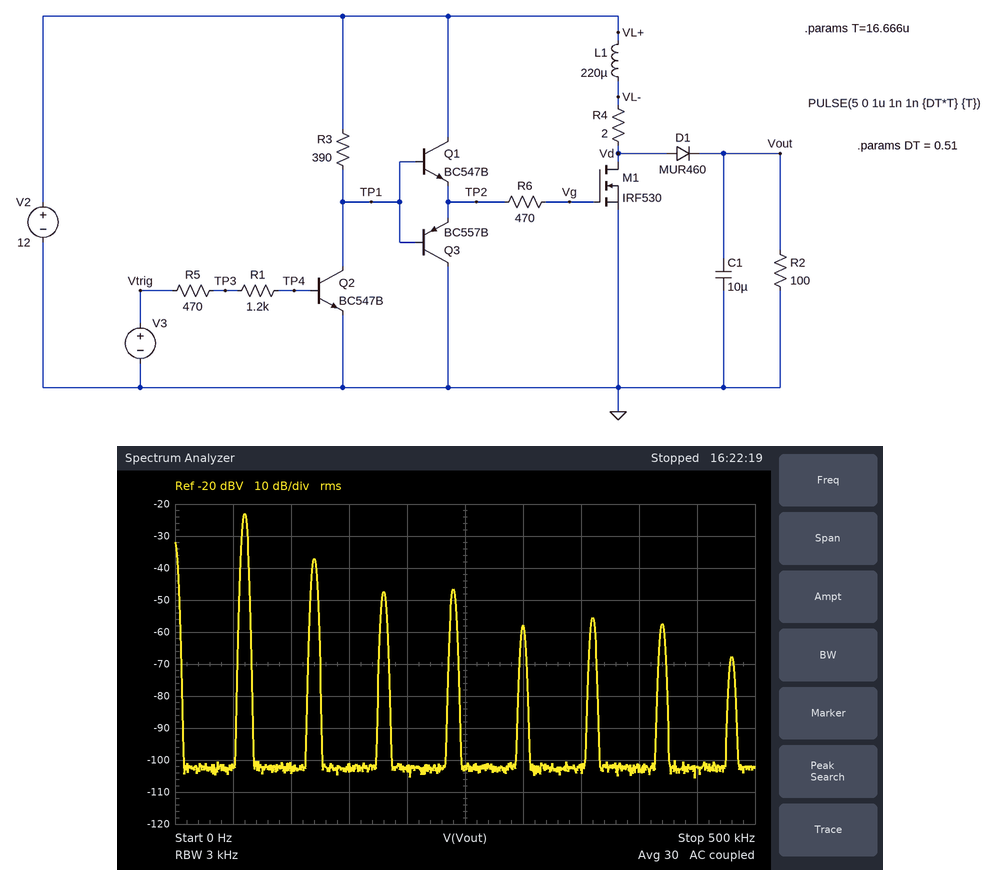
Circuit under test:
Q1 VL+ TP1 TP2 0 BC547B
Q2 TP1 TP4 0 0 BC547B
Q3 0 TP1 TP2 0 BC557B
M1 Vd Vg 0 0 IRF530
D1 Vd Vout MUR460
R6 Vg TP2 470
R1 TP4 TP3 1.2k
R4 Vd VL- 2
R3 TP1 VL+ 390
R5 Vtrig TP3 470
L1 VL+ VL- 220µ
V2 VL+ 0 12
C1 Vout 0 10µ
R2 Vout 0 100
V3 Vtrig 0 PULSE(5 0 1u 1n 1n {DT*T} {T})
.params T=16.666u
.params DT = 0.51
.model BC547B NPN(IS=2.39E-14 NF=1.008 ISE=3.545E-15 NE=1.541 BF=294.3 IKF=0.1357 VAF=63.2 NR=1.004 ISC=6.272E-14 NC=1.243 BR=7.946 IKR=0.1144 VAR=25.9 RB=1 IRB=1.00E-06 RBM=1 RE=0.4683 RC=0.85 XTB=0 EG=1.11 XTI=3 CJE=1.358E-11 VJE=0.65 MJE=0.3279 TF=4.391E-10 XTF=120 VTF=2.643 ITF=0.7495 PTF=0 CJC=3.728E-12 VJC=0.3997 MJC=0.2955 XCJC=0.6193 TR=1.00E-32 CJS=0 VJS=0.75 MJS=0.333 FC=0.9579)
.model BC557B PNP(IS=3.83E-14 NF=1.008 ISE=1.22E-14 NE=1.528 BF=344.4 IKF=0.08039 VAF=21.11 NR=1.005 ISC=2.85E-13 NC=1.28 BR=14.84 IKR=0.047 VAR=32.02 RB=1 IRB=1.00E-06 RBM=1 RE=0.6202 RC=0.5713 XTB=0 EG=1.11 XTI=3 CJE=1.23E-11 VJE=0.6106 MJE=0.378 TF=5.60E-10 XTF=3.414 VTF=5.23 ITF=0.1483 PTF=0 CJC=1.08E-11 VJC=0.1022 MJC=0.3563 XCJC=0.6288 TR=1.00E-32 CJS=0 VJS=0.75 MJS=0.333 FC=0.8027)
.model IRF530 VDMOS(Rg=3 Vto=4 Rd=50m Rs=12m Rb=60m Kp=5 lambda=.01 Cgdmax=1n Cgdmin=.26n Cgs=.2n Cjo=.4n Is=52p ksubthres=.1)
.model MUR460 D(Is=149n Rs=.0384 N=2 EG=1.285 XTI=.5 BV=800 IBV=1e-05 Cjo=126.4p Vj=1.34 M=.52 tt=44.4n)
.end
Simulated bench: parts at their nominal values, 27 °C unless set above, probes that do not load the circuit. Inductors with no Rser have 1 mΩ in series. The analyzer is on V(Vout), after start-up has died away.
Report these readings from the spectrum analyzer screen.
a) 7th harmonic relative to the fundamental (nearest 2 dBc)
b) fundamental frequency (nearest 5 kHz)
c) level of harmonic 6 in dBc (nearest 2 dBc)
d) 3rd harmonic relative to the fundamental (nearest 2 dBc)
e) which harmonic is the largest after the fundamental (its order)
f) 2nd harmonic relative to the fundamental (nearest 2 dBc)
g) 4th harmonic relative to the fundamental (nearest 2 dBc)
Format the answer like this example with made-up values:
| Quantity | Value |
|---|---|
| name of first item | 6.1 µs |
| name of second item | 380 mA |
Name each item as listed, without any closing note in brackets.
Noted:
| Quantity | Value |
|---|---|
| 7th harmonic relative to the fundamental | -34 dBc |
| fundamental frequency | 60 kHz |
| level of harmonic 6 in dBc | -32 dBc |
| 3rd harmonic relative to the fundamental | -24 dBc |
| which harmonic is the largest after the fundamental | 2 |
| 2nd harmonic relative to the fundamental | -14 dBc |
| 4th harmonic relative to the fundamental | -24 dBc |
